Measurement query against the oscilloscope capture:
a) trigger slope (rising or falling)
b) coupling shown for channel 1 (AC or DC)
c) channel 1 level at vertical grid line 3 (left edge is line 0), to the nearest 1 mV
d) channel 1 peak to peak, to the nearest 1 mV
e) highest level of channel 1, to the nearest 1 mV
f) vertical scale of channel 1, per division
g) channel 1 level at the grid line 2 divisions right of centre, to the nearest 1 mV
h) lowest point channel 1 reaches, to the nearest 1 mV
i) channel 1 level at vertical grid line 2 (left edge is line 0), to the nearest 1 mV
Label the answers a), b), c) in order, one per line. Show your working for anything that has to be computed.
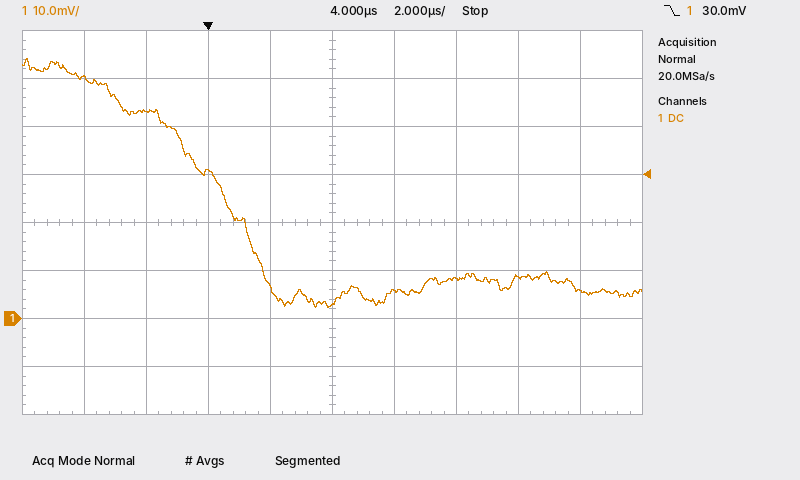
a) falling
b) DC
c) 31 mV
d) 54 mV − (2 mV) = 52 mV
e) 54 mV
f) 10 mV
g) 8 mV
h) 2 mV
i) 43 mV
